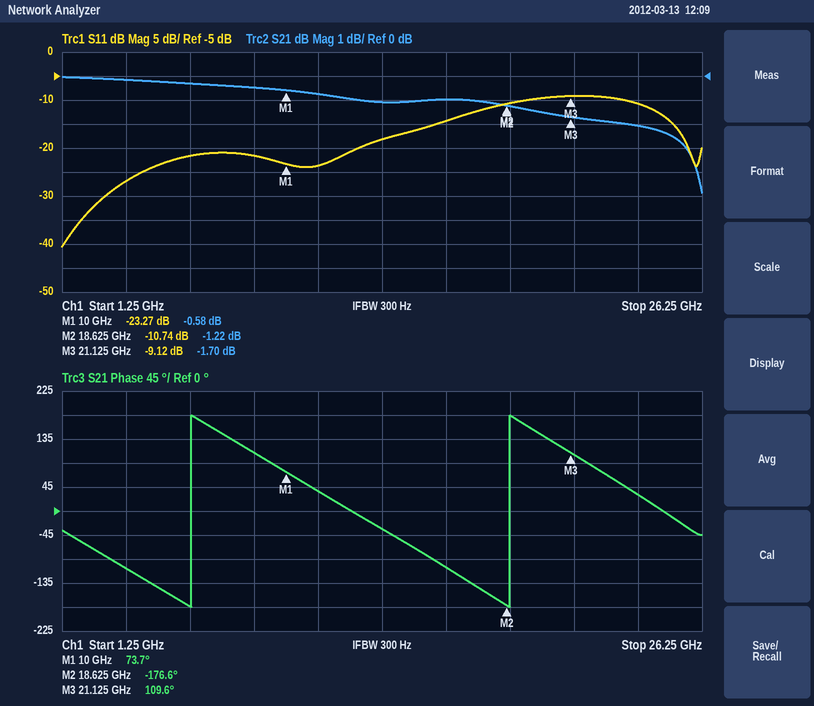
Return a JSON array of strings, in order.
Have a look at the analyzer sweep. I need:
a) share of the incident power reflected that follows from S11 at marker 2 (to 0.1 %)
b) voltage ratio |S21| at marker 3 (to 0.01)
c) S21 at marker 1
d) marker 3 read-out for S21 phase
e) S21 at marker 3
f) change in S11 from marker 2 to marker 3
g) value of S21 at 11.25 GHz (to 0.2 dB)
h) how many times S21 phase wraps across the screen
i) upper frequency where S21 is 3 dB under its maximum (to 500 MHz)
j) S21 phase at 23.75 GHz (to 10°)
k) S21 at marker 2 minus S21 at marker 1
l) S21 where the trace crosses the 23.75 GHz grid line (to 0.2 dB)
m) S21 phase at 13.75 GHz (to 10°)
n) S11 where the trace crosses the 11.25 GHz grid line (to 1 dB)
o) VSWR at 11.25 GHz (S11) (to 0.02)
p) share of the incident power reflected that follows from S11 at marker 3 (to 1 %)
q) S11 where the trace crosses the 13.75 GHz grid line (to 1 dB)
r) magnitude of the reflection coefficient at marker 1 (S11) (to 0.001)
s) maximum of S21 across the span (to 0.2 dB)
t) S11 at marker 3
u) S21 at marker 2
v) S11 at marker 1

["8.4 %", "0.82", "-0.58 dB", "109.6°", "-1.70 dB", "1.62 dB", "-0.8 dB", "2", "25.5 GHz", "30°", "-0.64 dB", "-2.0 dB", "-30°", "-24 dB", "1.14", "12 %", "-18 dB", "0.069", "0.0 dB", "-9.12 dB", "-1.22 dB", "-23.27 dB"]
